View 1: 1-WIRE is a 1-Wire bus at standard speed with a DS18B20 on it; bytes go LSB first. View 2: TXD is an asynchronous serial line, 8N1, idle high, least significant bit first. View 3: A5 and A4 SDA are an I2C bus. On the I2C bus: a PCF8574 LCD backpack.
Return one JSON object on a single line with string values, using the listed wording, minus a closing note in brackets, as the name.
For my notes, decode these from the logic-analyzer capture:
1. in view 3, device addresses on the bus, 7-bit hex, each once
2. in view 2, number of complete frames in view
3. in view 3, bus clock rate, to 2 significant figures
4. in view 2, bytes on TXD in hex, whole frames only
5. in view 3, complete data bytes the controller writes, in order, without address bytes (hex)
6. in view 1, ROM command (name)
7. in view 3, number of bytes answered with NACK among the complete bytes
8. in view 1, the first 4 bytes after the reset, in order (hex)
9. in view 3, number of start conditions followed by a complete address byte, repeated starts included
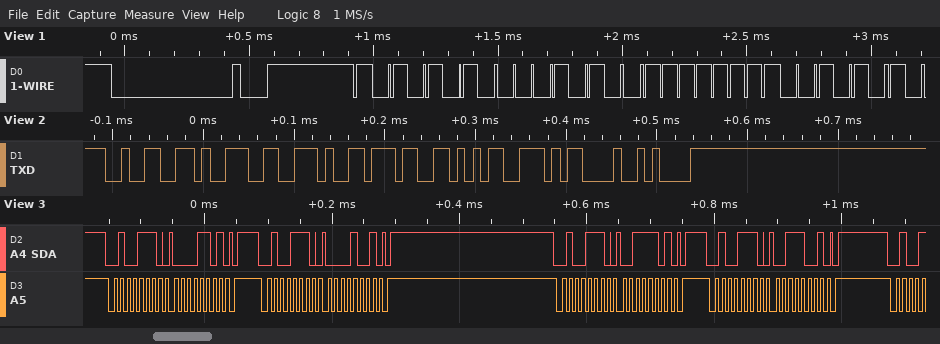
{"in view 3, device addresses on the bus, 7-bit hex, each once": "0x27", "in view 2, number of complete frames in view": "7", "in view 3, bus clock rate, to 2 significant figures": "100 kHz", "in view 2, bytes on TXD in hex, whole frames only": "0x32 0x39 0x2E 0x37 0x35 0x0D 0x0A", "in view 3, complete data bytes the controller writes, in order, without address bytes": "0D 09 3D 39", "in view 1, ROM command": "Match ROM", "in view 3, number of bytes answered with NACK among the complete bytes": "0", "in view 1, the first 4 bytes after the reset, in order": "55 28 FF 54", "in view 3, number of start conditions followed by a complete address byte, repeated starts included": "4"}
